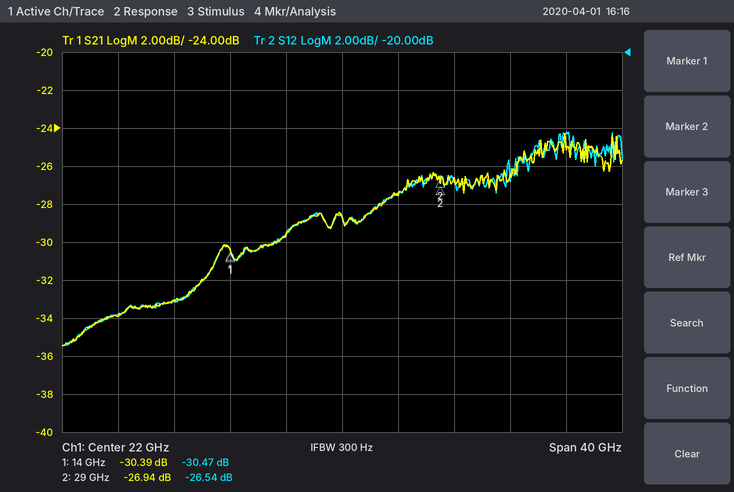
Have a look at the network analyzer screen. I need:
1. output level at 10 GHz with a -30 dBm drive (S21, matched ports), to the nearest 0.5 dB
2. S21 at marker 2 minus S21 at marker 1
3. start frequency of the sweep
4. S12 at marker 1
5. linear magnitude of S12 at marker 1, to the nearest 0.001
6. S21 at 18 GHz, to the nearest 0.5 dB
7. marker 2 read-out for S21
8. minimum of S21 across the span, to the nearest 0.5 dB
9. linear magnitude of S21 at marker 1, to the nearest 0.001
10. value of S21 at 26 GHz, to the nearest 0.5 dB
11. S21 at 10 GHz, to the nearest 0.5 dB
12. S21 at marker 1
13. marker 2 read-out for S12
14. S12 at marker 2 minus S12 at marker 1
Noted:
-63.0 dBm
3.45 dB
2 GHz
-30.47 dB
0.030
-29.5 dB
-26.94 dB
-35.5 dB
0.030
-27.5 dB
-33.0 dB
-30.39 dB
-26.54 dB
3.93 dB
